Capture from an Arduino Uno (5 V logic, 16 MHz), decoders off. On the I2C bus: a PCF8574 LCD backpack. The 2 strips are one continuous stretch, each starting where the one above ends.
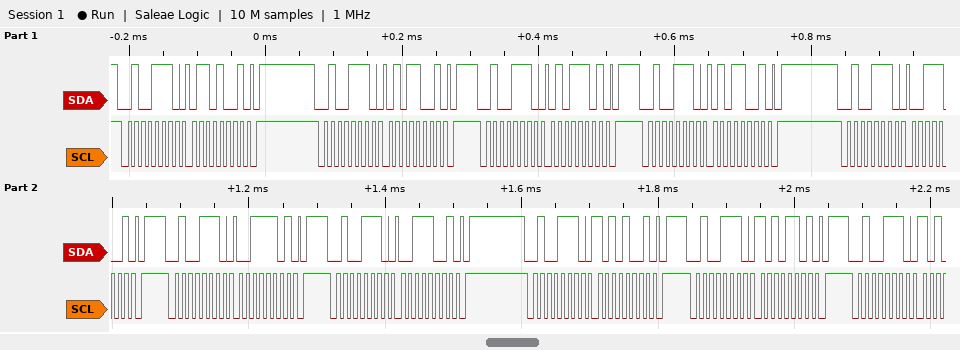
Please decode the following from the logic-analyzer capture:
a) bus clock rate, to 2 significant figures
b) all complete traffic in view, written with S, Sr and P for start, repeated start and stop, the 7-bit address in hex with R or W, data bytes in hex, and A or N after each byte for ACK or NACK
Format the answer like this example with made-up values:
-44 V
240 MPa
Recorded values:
100 kHz
S 27W A 69 A P S 27W A 59 A P S 27W A 5D A P S 27W A 59 A P S 27W A 39 A P S 27W A 3D A P S 27W A 39 A P S 27W A A9 A P S 27W A AD A P S 27W A
